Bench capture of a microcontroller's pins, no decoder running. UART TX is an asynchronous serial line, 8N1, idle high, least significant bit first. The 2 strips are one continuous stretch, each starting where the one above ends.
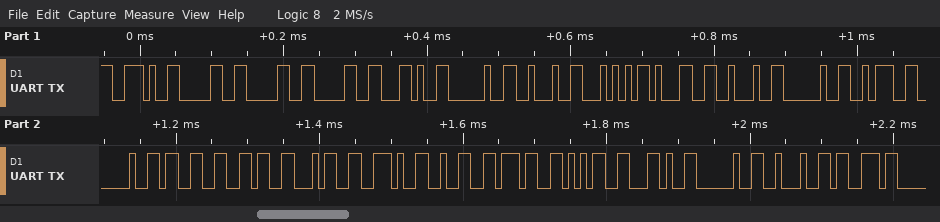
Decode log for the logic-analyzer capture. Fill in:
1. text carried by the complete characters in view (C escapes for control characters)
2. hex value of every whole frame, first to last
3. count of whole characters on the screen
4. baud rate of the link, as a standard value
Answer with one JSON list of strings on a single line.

["\".000, \\\"T1\\\" : 364.275, \\\"s\"", "2E 30 30 30 2C 20 22 54 31 22 20 3A 20 33 36 34 2E 32 37 35 2C 20 22 73", "24", "115200 baud"]
